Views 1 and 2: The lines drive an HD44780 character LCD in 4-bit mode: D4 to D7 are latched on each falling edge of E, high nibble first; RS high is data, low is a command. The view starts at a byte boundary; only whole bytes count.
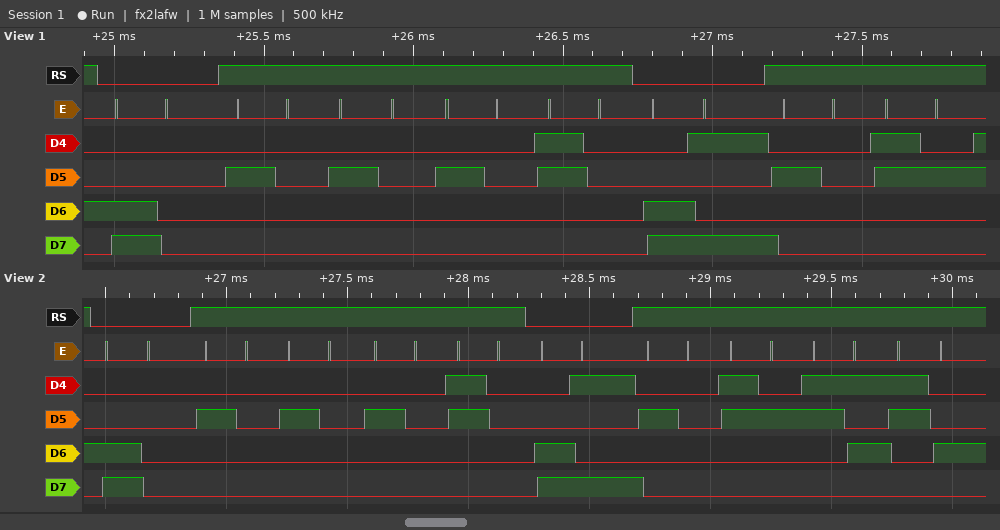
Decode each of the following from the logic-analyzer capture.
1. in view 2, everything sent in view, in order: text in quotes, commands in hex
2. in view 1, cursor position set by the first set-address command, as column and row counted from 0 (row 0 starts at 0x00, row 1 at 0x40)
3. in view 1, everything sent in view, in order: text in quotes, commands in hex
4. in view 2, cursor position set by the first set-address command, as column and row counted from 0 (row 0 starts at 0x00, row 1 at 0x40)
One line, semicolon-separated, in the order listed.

0xC0 "   0" 0xC9 " 254"; column 0, row 1; 0xC0 "   0" 0xC9 " 2"; column 0, row 1
